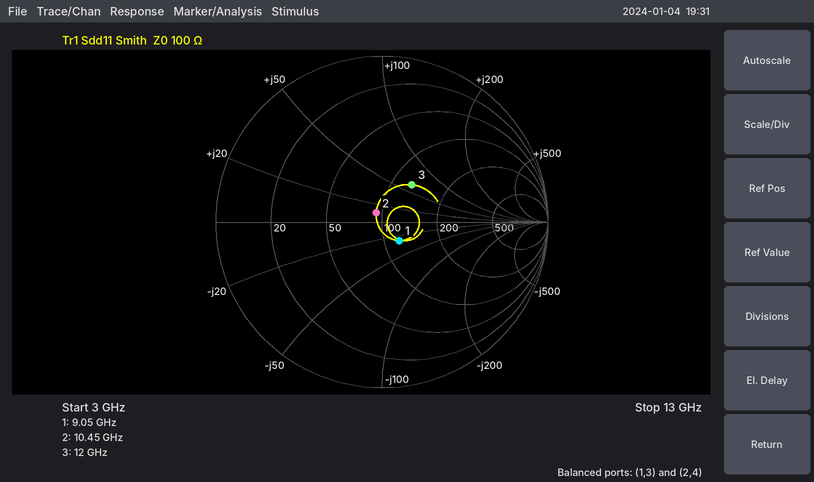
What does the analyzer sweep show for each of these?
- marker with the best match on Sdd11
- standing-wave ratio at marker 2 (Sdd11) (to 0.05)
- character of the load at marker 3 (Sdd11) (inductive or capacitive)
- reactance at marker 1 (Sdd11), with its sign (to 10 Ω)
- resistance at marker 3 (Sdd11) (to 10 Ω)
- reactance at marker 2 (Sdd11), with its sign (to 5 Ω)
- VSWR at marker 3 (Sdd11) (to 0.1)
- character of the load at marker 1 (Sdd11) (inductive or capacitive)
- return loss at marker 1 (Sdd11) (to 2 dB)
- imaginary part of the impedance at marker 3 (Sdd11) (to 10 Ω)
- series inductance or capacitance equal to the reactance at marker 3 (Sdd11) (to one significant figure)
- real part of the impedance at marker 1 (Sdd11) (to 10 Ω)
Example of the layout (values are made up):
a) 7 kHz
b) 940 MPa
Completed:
a) marker 2
b) 1.15
c) inductive
d) -30 Ω
e) 130 Ω
f) +10 Ω
g) 1.8
h) capacitive
i) 16 dB
j) +60 Ω
k) 800 pH
l) 120 Ω
